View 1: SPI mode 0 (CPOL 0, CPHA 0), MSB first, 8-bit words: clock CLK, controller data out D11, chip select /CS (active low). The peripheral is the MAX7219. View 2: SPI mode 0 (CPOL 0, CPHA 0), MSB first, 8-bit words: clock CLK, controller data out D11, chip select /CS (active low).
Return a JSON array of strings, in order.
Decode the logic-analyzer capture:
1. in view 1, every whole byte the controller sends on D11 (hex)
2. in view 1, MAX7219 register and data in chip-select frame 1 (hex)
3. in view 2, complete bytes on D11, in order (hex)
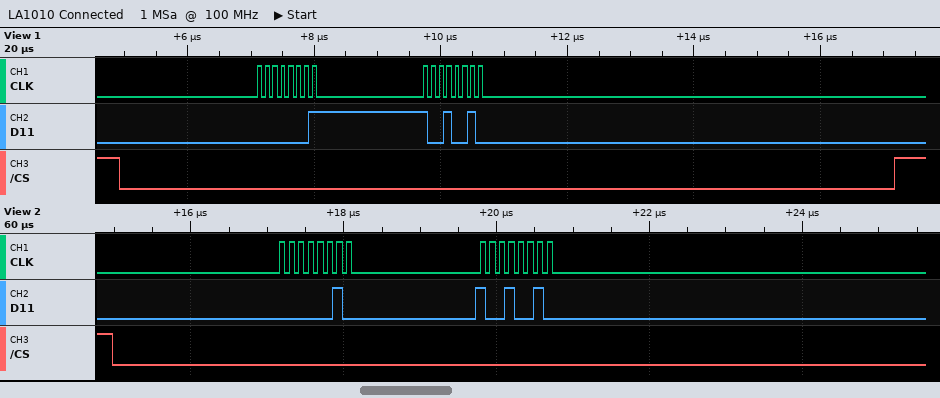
["0x01 0x92", "register 0x1, data 0x92", "02 92"]
